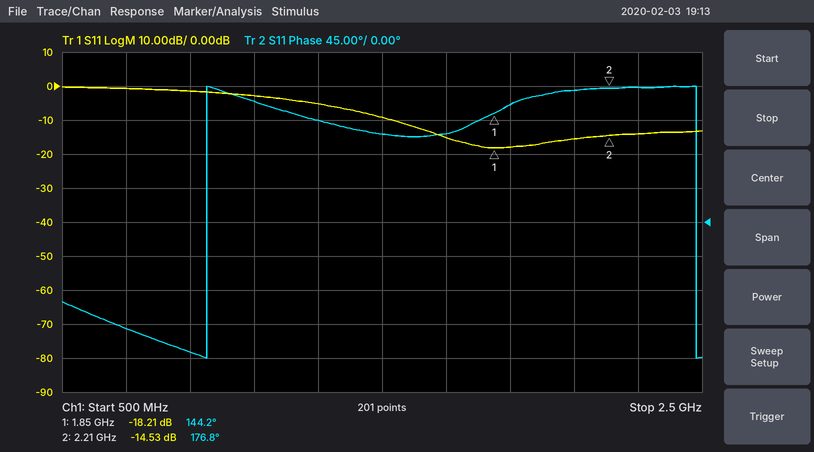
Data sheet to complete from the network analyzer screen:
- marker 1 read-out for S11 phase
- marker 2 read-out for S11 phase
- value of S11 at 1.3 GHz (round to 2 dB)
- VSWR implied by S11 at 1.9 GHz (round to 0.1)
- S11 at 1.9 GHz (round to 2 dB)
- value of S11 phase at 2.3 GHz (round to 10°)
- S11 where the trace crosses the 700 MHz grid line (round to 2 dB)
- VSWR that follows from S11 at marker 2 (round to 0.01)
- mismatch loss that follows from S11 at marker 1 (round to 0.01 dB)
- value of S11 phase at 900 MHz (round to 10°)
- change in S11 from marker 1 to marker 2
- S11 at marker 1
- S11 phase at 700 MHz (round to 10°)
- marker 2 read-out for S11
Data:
144.2°
176.8°
-6 dB
1.3
-18 dB
180°
0 dB
1.46
0.07 dB
-170°
3.68 dB
-18.21 dB
-140°
-14.53 dB
